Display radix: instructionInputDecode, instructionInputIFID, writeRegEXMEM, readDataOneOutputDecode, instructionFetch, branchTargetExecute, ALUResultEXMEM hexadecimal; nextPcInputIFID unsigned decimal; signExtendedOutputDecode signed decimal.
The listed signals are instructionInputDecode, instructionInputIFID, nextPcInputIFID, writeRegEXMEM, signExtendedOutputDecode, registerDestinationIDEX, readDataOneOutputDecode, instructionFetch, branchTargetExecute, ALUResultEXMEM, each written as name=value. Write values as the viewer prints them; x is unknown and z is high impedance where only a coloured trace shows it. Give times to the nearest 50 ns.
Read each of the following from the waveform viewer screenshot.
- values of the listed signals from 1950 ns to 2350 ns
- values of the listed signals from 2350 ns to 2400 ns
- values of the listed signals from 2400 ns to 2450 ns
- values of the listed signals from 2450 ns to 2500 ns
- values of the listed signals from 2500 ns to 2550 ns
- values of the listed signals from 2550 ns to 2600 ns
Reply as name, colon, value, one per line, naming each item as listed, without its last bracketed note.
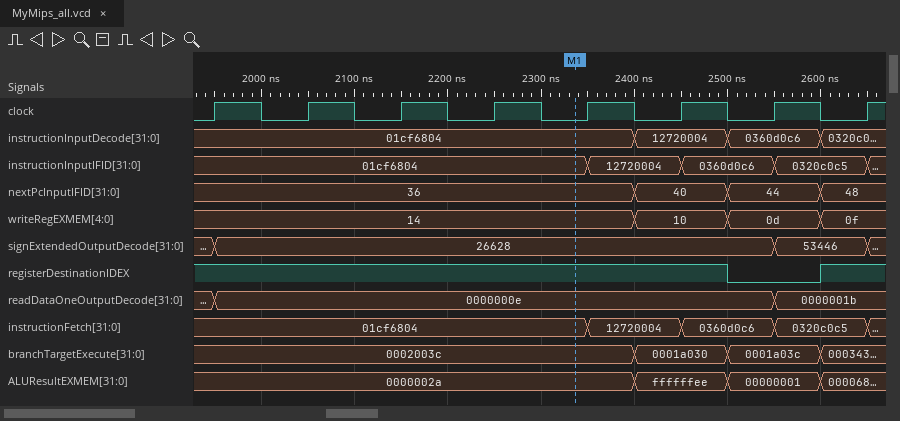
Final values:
values of the listed signals from 1950 ns to 2350 ns: instructionInputDecode=01cf6804, instructionInputIFID=01cf6804, nextPcInputIFID=36, writeRegEXMEM=14, signExtendedOutputDecode=26628, registerDestinationIDEX=1, readDataOneOutputDecode=0000000e, instructionFetch=01cf6804, branchTargetExecute=0002003c, ALUResultEXMEM=0000002a
values of the listed signals from 2350 ns to 2400 ns: instructionInputDecode=01cf6804, instructionInputIFID=12720004, nextPcInputIFID=36, writeRegEXMEM=14, signExtendedOutputDecode=26628, registerDestinationIDEX=1, readDataOneOutputDecode=0000000e, instructionFetch=12720004, branchTargetExecute=0002003c, ALUResultEXMEM=0000002a
values of the listed signals from 2400 ns to 2450 ns: instructionInputDecode=12720004, instructionInputIFID=12720004, nextPcInputIFID=40, writeRegEXMEM=10, signExtendedOutputDecode=26628, registerDestinationIDEX=1, readDataOneOutputDecode=0000000e, instructionFetch=12720004, branchTargetExecute=0001a030, ALUResultEXMEM=ffffffee
values of the listed signals from 2450 ns to 2500 ns: instructionInputDecode=12720004, instructionInputIFID=0360d0c6, nextPcInputIFID=40, writeRegEXMEM=10, signExtendedOutputDecode=26628, registerDestinationIDEX=1, readDataOneOutputDecode=0000000e, instructionFetch=0360d0c6, branchTargetExecute=0001a030, ALUResultEXMEM=ffffffee
values of the listed signals from 2500 ns to 2550 ns: instructionInputDecode=0360d0c6, instructionInputIFID=0360d0c6, nextPcInputIFID=44, writeRegEXMEM=0d, signExtendedOutputDecode=26628, registerDestinationIDEX=0, readDataOneOutputDecode=0000000e, instructionFetch=0360d0c6, branchTargetExecute=0001a03c, ALUResultEXMEM=00000001
values of the listed signals from 2550 ns to 2600 ns: instructionInputDecode=0360d0c6, instructionInputIFID=0320c0c5, nextPcInputIFID=44, writeRegEXMEM=0d, signExtendedOutputDecode=53446, registerDestinationIDEX=0, readDataOneOutputDecode=0000001b, instructionFetch=0320c0c5, branchTargetExecute=0001a03c, ALUResultEXMEM=00000001
